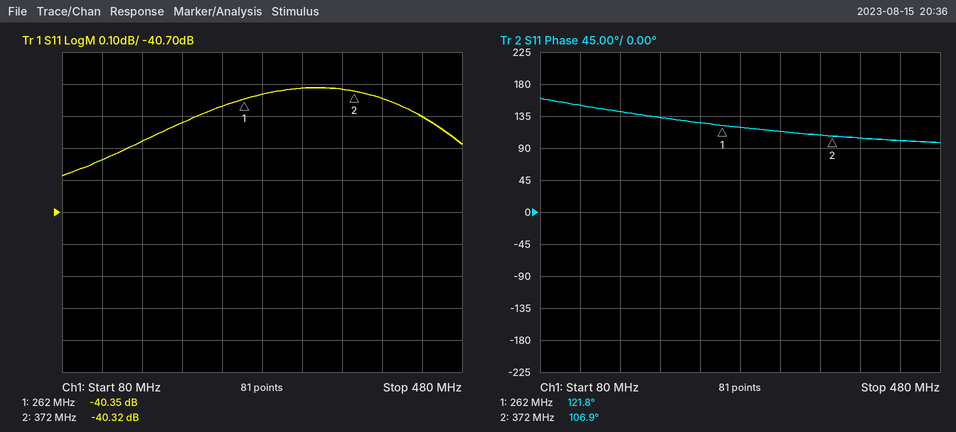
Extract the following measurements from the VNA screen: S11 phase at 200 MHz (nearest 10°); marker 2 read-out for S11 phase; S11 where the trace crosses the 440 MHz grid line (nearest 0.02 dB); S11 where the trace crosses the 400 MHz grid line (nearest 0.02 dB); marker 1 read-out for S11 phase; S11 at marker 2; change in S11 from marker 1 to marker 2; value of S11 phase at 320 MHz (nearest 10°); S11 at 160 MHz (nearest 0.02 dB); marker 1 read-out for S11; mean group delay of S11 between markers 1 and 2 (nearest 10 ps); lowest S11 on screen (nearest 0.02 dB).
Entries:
130°
106.9°
-40.40 dB
-40.34 dB
121.8°
-40.32 dB
0.03 dB
110°
-40.48 dB
-40.35 dB
380 ps
-40.58 dB
